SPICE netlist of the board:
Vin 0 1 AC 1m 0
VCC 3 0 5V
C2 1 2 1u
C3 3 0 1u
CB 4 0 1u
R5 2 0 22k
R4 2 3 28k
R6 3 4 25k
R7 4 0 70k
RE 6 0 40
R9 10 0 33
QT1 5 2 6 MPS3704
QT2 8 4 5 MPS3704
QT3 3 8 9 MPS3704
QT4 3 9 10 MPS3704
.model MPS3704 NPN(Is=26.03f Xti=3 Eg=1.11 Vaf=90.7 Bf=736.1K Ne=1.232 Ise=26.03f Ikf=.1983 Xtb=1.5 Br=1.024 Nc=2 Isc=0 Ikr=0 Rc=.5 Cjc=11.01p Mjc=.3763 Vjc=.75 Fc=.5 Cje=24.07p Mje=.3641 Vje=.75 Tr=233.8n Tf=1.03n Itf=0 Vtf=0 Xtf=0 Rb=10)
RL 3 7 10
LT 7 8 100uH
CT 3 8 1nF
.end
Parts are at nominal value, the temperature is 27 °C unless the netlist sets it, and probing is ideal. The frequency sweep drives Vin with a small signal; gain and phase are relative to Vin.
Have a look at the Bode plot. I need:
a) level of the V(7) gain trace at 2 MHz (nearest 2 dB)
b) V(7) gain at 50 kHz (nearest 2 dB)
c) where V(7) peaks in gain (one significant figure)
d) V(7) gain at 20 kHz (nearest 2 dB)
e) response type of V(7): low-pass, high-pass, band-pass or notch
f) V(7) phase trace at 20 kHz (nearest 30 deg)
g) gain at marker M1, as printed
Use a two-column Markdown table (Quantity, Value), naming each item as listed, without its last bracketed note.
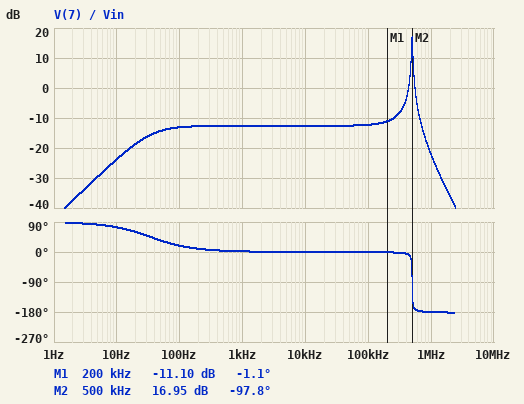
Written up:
| Quantity | Value |
|---|---|
| level of the V(7) gain trace at 2 MHz | -36 dB |
| V(7) gain at 50 kHz | -12 dB |
| where V(7) peaks in gain | 500 kHz |
| V(7) gain at 20 kHz | -12 dB |
| response type of V(7): low-pass, high-pass, band-pass or notch | band-pass |
| V(7) phase trace at 20 kHz | 0 deg |
| gain at marker M1, as printed | -11.10 dB |
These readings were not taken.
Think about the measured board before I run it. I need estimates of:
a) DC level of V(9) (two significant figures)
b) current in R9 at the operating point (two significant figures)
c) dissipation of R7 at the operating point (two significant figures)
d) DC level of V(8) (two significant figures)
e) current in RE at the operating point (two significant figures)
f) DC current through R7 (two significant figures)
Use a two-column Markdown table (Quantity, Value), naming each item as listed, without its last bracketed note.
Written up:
| Quantity | Value |
|---|---|
| DC level of V(9) | 4.3 V |
| current in R9 at the operating point | 110 mA |
| dissipation of R7 at the operating point | 70 µW |
| DC level of V(8) | 4.9 V |
| current in RE at the operating point | 12 mA |
| DC current through R7 | 32 µA |
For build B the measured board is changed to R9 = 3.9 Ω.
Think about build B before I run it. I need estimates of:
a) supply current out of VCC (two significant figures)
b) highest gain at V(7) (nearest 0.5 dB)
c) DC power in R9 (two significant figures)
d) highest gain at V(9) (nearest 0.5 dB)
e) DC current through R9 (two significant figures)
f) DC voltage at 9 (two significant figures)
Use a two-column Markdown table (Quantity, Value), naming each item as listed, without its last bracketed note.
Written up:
| Quantity | Value |
|---|---|
| supply current out of VCC | 850 mA |
| highest gain at V(7) | 15.5 dB |
| DC power in R9 | 2.7 W |
| highest gain at V(9) | 45.5 dB |
| DC current through R9 | 830 mA |
| DC voltage at 9 | 4.2 V |
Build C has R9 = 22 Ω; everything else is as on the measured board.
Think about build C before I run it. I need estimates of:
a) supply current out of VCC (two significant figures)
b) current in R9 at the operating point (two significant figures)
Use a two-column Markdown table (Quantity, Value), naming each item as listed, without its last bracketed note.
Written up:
| Quantity | Value |
|---|---|
| supply current out of VCC | 170 mA |
| current in R9 at the operating point | 160 mA |
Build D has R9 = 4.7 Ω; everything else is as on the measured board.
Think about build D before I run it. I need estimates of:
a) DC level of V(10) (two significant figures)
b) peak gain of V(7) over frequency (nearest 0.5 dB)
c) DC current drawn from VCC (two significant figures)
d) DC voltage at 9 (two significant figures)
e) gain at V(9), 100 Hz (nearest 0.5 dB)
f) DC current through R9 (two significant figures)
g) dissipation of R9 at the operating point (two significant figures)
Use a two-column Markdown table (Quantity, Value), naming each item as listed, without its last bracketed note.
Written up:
| Quantity | Value |
|---|---|
| DC level of V(10) | 3.3 V |
| peak gain of V(7) over frequency | 16.0 dB |
| DC current drawn from VCC | 710 mA |
| DC voltage at 9 | 4.2 V |
| gain at V(9), 100 Hz | -13.0 dB |
| DC current through R9 | 700 mA |
| dissipation of R9 at the operating point | 2.3 W |
